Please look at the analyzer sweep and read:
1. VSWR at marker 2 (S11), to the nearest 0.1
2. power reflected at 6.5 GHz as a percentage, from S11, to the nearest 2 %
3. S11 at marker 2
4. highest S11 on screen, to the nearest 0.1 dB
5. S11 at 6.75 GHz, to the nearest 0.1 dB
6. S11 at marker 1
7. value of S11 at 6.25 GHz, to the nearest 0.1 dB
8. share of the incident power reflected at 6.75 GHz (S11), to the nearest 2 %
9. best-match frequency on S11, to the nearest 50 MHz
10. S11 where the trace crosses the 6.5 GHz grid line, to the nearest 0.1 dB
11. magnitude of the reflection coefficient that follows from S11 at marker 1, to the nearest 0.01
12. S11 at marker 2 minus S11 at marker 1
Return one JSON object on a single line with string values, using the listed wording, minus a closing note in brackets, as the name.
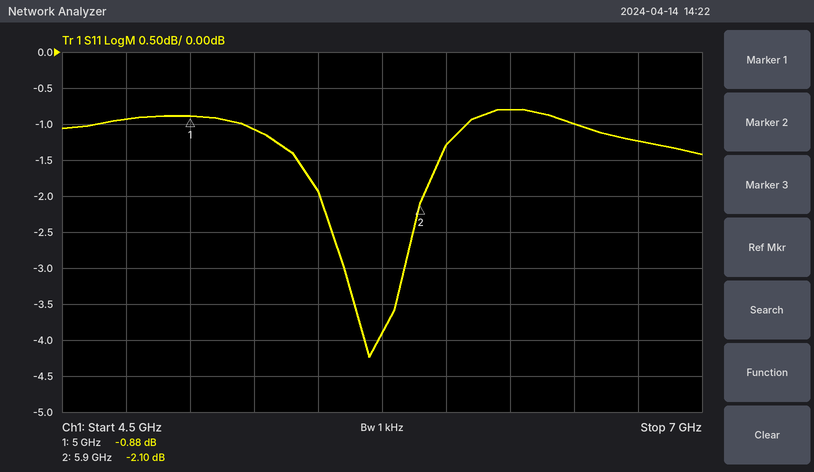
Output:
{"VSWR at marker 2 (S11), to the nearest 0.1": "8.3", "power reflected at 6.5 GHz as a percentage, from S11, to the nearest 2 %": "80 %", "S11 at marker 2": "-2.10 dB", "highest S11 on screen, to the nearest 0.1 dB": "-0.8 dB", "S11 at 6.75 GHz, to the nearest 0.1 dB": "-1.2 dB", "S11 at marker 1": "-0.88 dB", "value of S11 at 6.25 GHz, to the nearest 0.1 dB": "-0.8 dB", "share of the incident power reflected at 6.75 GHz (S11), to the nearest 2 %": "76 %", "best-match frequency on S11, to the nearest 50 MHz": "5.70 GHz", "S11 where the trace crosses the 6.5 GHz grid line, to the nearest 0.1 dB": "-1.0 dB", "magnitude of the reflection coefficient that follows from S11 at marker 1, to the nearest 0.01": "0.90", "S11 at marker 2 minus S11 at marker 1": "-1.22 dB"}
